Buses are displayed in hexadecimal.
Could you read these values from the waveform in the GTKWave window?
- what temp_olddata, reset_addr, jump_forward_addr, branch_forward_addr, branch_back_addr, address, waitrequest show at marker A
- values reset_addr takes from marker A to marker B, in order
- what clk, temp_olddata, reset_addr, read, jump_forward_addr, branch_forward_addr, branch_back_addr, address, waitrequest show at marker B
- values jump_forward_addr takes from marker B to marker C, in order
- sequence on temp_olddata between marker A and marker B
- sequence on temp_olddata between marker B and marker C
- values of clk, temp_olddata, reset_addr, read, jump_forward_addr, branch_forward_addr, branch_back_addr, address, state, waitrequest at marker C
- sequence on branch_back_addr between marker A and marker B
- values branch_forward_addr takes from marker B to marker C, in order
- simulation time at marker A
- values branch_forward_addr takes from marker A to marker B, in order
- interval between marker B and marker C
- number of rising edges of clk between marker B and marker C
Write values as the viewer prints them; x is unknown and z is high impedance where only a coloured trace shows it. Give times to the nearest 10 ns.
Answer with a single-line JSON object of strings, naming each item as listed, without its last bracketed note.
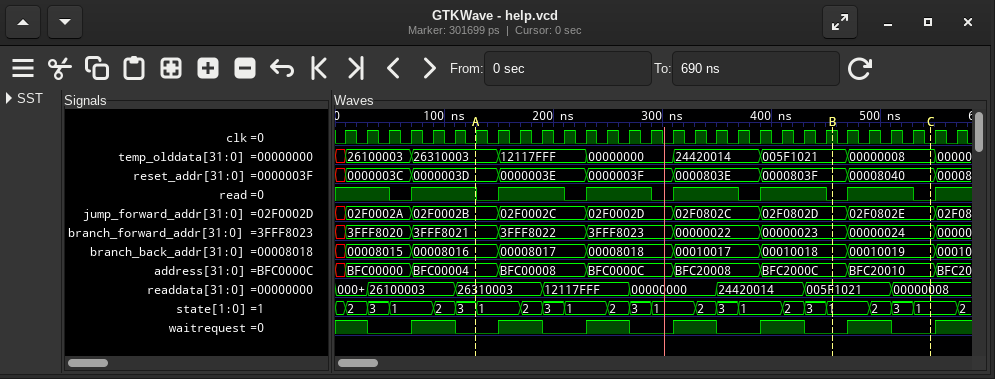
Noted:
{"what temp_olddata, reset_addr, jump_forward_addr, branch_forward_addr, branch_back_addr, address, waitrequest show at marker A": "temp_olddata=26310003, reset_addr=0000003D, jump_forward_addr=02F0002B, branch_forward_addr=3FFF8021, branch_back_addr=00008016, address=BFC00004, waitrequest=0", "values reset_addr takes from marker A to marker B, in order": "0000003D, 0000003E, 0000003F, 0000803E, 0000803F", "what clk, temp_olddata, reset_addr, read, jump_forward_addr, branch_forward_addr, branch_back_addr, address, waitrequest show at marker B": "clk=1, temp_olddata=005F1021, reset_addr=0000803F, read=0, jump_forward_addr=02F0802D, branch_forward_addr=00000023, branch_back_addr=00010018, address=BFC2000C, waitrequest=0", "values jump_forward_addr takes from marker B to marker C, in order": "02F0802D, 02F0802E", "sequence on temp_olddata between marker A and marker B": "26310003, 12117FFF, 00000000, 24420014, 005F1021", "sequence on temp_olddata between marker B and marker C": "005F1021, 00000008", "values of clk, temp_olddata, reset_addr, read, jump_forward_addr, branch_forward_addr, branch_back_addr, address, state, waitrequest at marker C": "clk=0, temp_olddata=00000008, reset_addr=00008040, read=0, jump_forward_addr=02F0802E, branch_forward_addr=00000024, branch_back_addr=00010019, address=BFC20010, state=1, waitrequest=0", "sequence on branch_back_addr between marker A and marker B": "00008016, 00008017, 00008018, 00010017, 00010018", "values branch_forward_addr takes from marker B to marker C, in order": "00000023, 00000024", "simulation time at marker A": "130 ns", "values branch_forward_addr takes from marker A to marker B, in order": "3FFF8021, 3FFF8022, 3FFF8023, 00000022, 00000023", "interval between marker B and marker C": "90 ns", "number of rising edges of clk between marker B and marker C": "4"}
